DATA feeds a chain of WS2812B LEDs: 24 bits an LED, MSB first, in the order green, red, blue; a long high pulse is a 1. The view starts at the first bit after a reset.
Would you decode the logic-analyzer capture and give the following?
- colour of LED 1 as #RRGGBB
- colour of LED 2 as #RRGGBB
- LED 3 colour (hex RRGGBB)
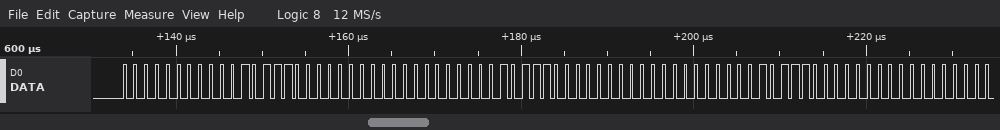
#170000
#170000
#170000
